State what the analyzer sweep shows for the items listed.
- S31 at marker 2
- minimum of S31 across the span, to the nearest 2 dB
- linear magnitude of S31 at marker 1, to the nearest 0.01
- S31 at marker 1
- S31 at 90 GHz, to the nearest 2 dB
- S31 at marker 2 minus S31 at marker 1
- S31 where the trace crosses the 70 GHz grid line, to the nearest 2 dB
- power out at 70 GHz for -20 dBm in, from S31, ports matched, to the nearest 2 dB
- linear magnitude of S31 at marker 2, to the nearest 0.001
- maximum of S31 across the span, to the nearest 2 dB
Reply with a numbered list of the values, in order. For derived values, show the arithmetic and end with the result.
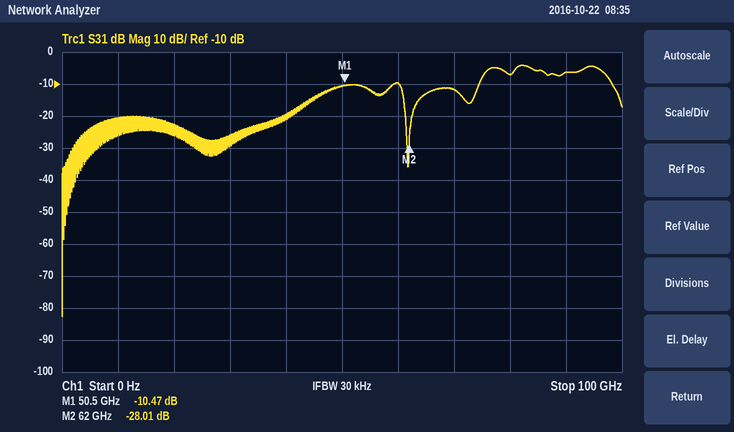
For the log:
1. -28.01 dB
2. -82 dB
3. 10^(-10.47/20) ≈ 0.30
4. -10.47 dB
5. -6 dB
6. -28.01 − (-10.47) = -17.54 dB
7. -12 dB
8. -20 dBm + (-12 dB) = -32 dBm
9. 10^(-28.01/20) ≈ 0.040
10. -4 dB
